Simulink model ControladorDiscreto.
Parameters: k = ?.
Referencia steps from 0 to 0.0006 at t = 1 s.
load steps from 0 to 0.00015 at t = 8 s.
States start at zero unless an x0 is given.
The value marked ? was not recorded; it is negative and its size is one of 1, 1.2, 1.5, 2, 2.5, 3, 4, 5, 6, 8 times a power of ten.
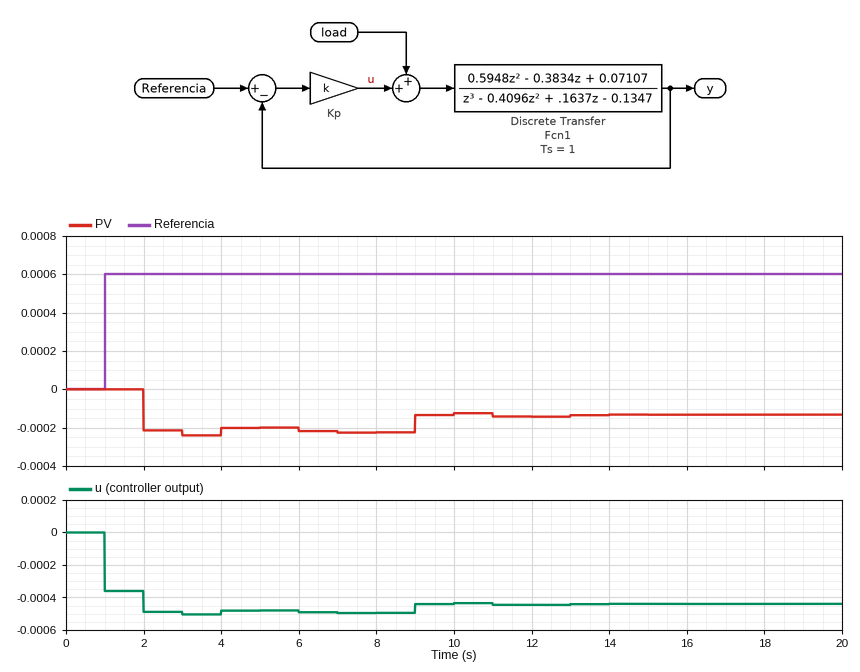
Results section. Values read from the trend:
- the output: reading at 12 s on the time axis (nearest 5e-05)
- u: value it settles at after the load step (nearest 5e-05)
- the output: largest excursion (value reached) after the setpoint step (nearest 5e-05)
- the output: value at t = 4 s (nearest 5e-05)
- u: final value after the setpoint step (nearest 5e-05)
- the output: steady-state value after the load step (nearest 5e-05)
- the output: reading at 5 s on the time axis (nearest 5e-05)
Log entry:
-0.00015
-0.00045
-0.00025
-0.00020
-0.00050
-0.00015
-0.00020
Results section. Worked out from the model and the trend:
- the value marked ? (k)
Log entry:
-0.6
